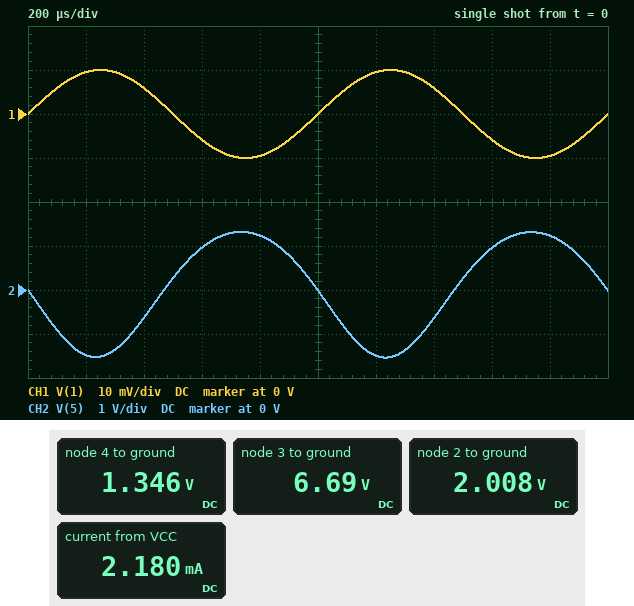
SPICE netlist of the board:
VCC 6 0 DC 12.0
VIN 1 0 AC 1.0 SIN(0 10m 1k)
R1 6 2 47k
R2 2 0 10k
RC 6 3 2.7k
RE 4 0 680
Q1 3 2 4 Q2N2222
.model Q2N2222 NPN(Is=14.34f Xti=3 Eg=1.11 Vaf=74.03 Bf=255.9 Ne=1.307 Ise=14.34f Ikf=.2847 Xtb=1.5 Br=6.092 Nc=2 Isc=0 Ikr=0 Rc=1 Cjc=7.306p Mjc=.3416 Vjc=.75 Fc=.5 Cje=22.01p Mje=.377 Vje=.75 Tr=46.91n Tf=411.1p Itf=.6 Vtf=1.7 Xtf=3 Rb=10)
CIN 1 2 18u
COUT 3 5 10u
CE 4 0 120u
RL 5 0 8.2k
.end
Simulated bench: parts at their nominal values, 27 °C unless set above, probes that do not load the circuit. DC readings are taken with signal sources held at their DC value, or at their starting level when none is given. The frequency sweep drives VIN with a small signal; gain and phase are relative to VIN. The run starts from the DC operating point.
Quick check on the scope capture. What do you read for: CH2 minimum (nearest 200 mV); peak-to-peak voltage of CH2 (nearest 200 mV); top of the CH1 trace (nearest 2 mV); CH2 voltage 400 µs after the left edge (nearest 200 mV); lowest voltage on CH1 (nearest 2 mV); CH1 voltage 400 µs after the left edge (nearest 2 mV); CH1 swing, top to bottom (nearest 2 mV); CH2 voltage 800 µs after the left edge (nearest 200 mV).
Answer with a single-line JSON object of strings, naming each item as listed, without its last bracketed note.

{"CH2 minimum": "-1.6 V", "peak-to-peak voltage of CH2": "2.8 V", "top of the CH1 trace": "10 mV", "CH2 voltage 400 µs after the left edge": "-600 mV", "lowest voltage on CH1": "-10 mV", "CH1 voltage 400 µs after the left edge": "6 mV", "CH1 swing, top to bottom": "20 mV", "CH2 voltage 800 µs after the left edge": "1.2 V"}
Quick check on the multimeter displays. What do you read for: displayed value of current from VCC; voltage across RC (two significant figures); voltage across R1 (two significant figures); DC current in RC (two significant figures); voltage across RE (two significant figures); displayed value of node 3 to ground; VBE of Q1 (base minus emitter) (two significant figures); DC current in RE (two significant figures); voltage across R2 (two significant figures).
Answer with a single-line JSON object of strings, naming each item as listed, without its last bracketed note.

{"displayed value of current from VCC": "2.180 mA", "voltage across RC": "5.3 V", "voltage across R1": "10 V", "DC current in RC": "2.0 mA", "voltage across RE": "1.3 V", "displayed value of node 3 to ground": "6.69 V", "VBE of Q1 (base minus emitter)": "660 mV", "DC current in RE": "2.0 mA", "voltage across R2": "2.0 V"}
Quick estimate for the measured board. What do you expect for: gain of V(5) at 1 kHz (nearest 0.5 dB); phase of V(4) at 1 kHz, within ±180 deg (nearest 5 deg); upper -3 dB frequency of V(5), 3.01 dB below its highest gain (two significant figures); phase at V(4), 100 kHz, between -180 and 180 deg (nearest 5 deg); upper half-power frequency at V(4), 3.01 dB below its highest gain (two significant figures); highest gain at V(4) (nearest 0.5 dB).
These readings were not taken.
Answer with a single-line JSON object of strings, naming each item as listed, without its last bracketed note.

{"gain of V(5) at 1 kHz": "43.0 dB", "phase of V(4) at 1 kHz, within ±180 deg": "-85 deg", "upper -3 dB frequency of V(5), 3.01 dB below its highest gain": "12 MHz", "phase at V(4), 100 kHz, between -180 and 180 deg": "-90 deg", "upper half-power frequency at V(4), 3.01 dB below its highest gain": "100 Hz", "highest gain at V(4)": "-0.5 dB"}
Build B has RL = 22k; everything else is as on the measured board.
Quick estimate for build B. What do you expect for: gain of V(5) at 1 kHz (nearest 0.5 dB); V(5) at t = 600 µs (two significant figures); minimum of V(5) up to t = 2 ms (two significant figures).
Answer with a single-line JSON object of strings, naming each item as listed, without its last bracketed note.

{"gain of V(5) at 1 kHz": "44.5 dB", "V(5) at t = 600 µs": "1.1 V", "minimum of V(5) up to t = 2 ms": "-1.8 V"}
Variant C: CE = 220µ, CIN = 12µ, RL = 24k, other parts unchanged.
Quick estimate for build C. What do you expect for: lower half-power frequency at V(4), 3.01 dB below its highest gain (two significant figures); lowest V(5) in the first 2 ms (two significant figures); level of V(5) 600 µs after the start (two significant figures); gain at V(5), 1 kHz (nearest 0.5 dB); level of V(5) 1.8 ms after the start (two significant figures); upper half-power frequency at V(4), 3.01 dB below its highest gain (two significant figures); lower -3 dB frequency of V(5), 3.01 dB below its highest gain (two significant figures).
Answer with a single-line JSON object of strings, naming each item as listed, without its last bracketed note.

{"lower half-power frequency at V(4), 3.01 dB below its highest gain": "1.5 Hz", "lowest V(5) in the first 2 ms": "-1.9 V", "level of V(5) 600 µs after the start": "1.1 V", "gain at V(5), 1 kHz": "44.5 dB", "level of V(5) 1.8 ms after the start": "1.5 V", "upper half-power frequency at V(4), 3.01 dB below its highest gain": "61 Hz", "lower -3 dB frequency of V(5), 3.01 dB below its highest gain": "58 Hz"}
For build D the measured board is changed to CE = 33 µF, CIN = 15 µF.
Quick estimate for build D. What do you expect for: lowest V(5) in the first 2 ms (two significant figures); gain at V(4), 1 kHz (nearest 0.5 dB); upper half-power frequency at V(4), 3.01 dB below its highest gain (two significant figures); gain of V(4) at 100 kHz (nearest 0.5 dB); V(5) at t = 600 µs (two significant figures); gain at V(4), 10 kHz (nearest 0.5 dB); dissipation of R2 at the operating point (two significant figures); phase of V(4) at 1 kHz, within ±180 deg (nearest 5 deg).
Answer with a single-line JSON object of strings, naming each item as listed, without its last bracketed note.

{"lowest V(5) in the first 2 ms": "-1.4 V", "gain at V(4), 1 kHz": "-9.5 dB", "upper half-power frequency at V(4), 3.01 dB below its highest gain": "360 Hz", "gain of V(4) at 100 kHz": "-49.0 dB", "V(5) at t = 600 µs": "1.1 V", "gain at V(4), 10 kHz": "-29.0 dB", "dissipation of R2 at the operating point": "400 µW", "phase of V(4) at 1 kHz, within ±180 deg": "-70 deg"}
